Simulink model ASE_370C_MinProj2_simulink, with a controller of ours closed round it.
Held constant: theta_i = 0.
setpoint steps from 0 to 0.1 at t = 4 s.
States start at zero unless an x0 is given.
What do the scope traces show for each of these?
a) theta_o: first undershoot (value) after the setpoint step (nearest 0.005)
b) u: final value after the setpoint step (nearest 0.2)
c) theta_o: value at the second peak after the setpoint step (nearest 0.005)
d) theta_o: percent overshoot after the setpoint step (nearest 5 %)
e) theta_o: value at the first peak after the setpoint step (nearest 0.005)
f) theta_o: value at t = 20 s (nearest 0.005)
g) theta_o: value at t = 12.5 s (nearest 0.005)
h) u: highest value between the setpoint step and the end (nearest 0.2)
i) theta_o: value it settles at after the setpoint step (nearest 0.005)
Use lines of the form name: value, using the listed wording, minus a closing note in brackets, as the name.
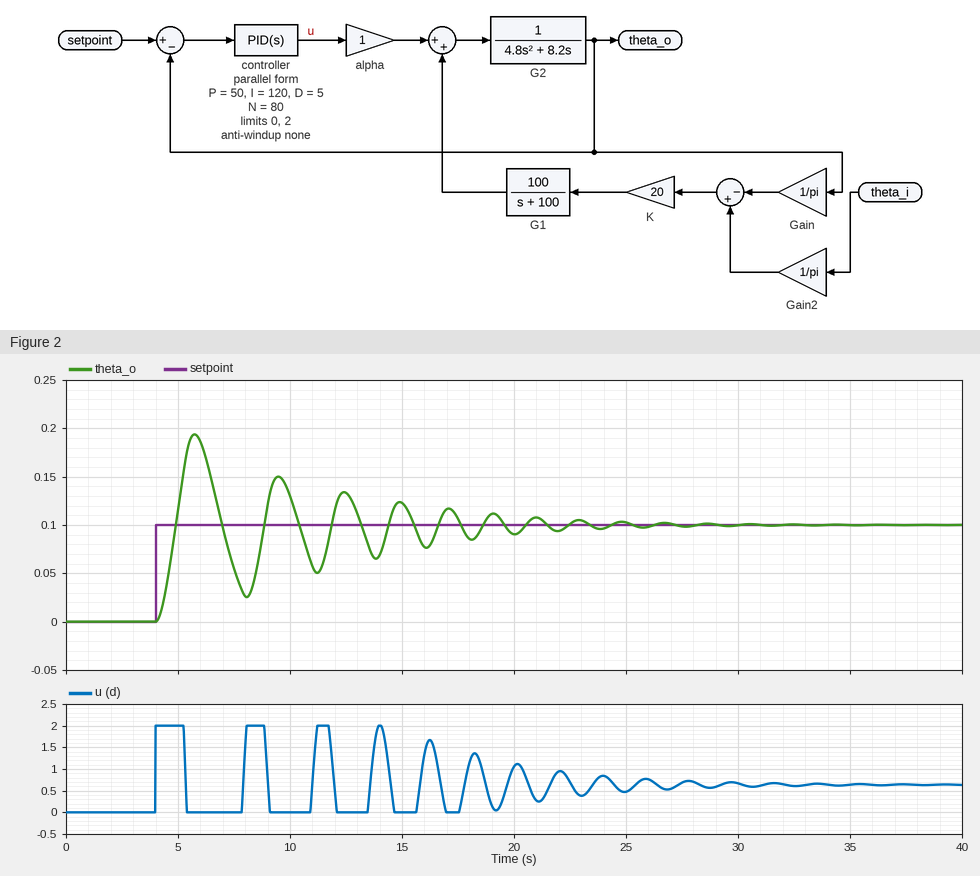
theta_o: first undershoot (value) after the setpoint step: 0.025
u: final value after the setpoint step: 0.6
theta_o: value at the second peak after the setpoint step: 0.150
theta_o: percent overshoot after the setpoint step: 95 %
theta_o: value at the first peak after the setpoint step: 0.195
theta_o: value at t = 20 s: 0.090
theta_o: value at t = 12.5 s: 0.135
u: highest value between the setpoint step and the end: 2.0
theta_o: value it settles at after the setpoint step: 0.100
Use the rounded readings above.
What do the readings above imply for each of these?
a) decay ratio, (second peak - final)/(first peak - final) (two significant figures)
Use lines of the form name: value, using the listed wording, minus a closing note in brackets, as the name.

decay ratio, (second peak - final)/(first peak - final): 0.53
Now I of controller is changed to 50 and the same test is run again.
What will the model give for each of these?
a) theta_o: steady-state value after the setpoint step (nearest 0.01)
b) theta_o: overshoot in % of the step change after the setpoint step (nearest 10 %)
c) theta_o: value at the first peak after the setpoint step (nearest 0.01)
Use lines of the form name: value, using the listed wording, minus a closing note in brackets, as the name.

theta_o: steady-state value after the setpoint step: 0.10
theta_o: overshoot in % of the step change after the setpoint step: 60 %
theta_o: value at the first peak after the setpoint step: 0.16
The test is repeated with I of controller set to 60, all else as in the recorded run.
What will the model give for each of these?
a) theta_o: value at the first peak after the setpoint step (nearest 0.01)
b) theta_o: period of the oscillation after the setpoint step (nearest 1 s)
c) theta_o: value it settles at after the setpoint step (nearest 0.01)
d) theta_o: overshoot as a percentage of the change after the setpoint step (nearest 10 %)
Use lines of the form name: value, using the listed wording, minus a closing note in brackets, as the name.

theta_o: value at the first peak after the setpoint step: 0.16
theta_o: period of the oscillation after the setpoint step: 3 s
theta_o: value it settles at after the setpoint step: 0.10
theta_o: overshoot as a percentage of the change after the setpoint step: 60 %
